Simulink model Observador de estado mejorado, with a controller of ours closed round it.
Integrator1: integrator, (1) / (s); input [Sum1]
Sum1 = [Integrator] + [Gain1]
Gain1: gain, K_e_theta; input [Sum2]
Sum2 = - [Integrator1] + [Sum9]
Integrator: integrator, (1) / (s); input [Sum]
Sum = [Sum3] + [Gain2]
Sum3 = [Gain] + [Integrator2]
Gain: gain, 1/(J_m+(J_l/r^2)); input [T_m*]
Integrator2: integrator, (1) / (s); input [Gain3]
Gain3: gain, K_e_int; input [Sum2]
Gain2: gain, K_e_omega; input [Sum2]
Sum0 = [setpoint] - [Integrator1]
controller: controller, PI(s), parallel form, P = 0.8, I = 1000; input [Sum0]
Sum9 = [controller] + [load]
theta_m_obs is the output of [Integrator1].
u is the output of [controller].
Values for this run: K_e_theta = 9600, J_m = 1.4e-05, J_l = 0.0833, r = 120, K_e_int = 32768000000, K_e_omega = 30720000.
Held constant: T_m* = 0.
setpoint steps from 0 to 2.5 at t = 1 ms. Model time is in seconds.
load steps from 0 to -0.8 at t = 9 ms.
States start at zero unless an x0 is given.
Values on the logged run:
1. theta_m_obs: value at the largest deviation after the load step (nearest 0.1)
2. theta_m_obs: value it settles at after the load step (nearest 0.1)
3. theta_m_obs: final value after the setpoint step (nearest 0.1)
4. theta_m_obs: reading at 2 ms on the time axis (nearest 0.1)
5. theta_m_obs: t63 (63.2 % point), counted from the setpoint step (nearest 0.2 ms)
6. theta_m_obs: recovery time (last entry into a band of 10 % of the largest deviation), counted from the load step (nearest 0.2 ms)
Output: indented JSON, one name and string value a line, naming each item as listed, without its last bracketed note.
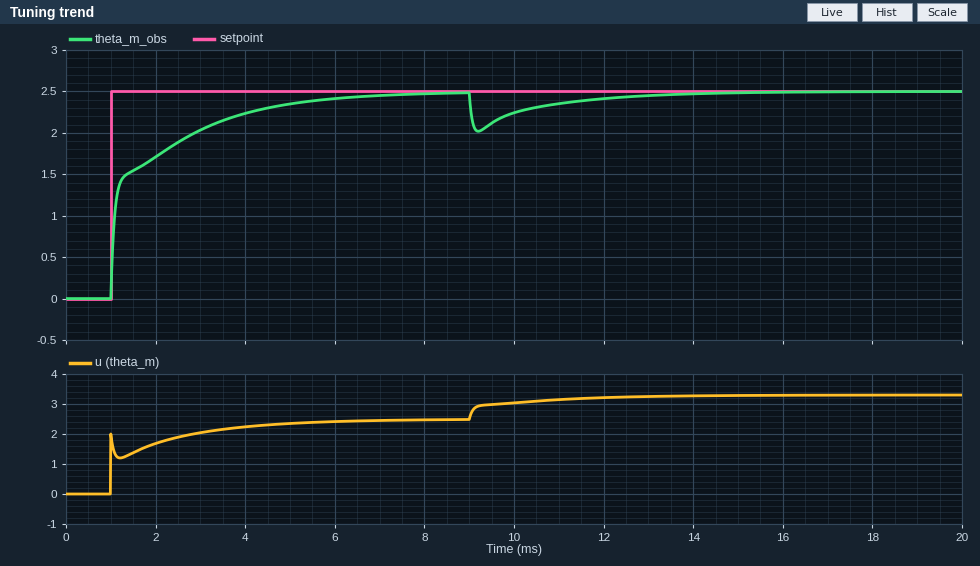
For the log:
{
  "theta_m_obs: value at the largest deviation after the load step": "2.0",
  "theta_m_obs: value it settles at after the load step": "2.5",
  "theta_m_obs: final value after the setpoint step": "2.5",
  "theta_m_obs: reading at 2 ms on the time axis": "1.7",
  "theta_m_obs: t63 (63.2 % point), counted from the setpoint step": "0.6 ms",
  "theta_m_obs: recovery time (last entry into a band of 10 % of the largest deviation), counted from the load step": "4.2 ms"
}
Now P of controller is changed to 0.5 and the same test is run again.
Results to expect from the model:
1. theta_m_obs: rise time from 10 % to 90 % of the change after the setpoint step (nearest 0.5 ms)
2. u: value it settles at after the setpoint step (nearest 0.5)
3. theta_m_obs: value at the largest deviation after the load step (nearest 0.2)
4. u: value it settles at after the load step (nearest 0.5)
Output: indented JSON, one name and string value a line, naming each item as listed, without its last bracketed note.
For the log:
{
  "theta_m_obs: rise time from 10 % to 90 % of the change after the setpoint step": "3.0 ms",
  "u: value it settles at after the setpoint step": "2.5",
  "theta_m_obs: value at the largest deviation after the load step": "2.0",
  "u: value it settles at after the load step": "3.5"
}
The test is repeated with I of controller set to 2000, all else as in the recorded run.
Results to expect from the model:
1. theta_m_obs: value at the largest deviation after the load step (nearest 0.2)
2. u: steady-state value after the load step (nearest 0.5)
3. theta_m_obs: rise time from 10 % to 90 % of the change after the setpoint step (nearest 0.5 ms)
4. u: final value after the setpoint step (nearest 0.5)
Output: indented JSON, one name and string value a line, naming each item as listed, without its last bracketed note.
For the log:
{
  "theta_m_obs: value at the largest deviation after the load step": "2.0",
  "u: steady-state value after the load step": "3.5",
  "theta_m_obs: rise time from 10 % to 90 % of the change after the setpoint step": "1.5 ms",
  "u: final value after the setpoint step": "2.5"
}
